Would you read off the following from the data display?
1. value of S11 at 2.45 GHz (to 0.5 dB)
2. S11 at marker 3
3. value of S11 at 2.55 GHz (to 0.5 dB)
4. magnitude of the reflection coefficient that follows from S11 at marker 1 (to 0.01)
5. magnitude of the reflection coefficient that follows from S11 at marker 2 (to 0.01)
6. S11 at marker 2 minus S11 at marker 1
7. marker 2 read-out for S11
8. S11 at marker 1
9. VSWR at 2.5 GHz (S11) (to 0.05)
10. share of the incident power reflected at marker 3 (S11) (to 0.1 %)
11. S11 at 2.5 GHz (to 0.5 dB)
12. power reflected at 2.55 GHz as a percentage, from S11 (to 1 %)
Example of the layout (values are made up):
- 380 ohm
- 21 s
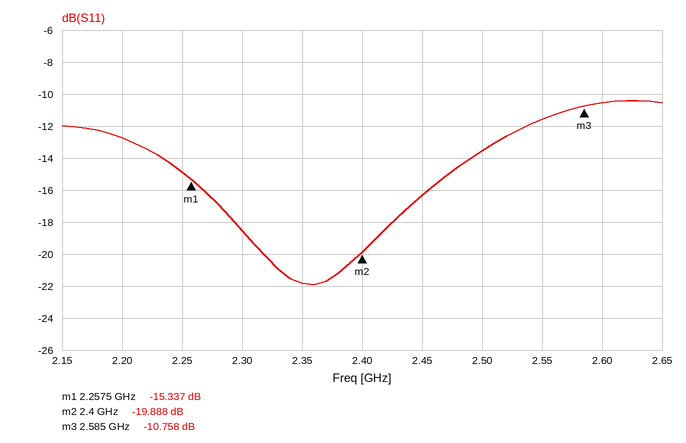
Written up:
- -16.5 dB
- -10.758 dB
- -11.5 dB
- 0.17
- 0.10
- -4.551 dB
- -19.888 dB
- -15.337 dB
- 1.55
- 8.4 %
- -13.5 dB
- 7 %
